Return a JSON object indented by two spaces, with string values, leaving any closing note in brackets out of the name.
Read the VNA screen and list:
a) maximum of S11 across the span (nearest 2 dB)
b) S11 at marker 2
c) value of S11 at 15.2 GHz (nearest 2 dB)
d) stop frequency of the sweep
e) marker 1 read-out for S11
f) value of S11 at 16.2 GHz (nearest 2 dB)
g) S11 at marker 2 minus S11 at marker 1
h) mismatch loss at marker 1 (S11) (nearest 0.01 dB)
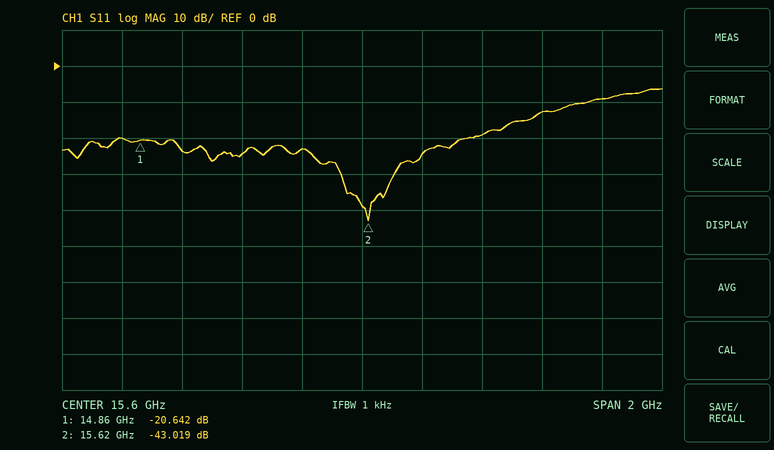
{
  "maximum of S11 across the span": "-6 dB",
  "S11 at marker 2": "-43.019 dB",
  "value of S11 at 15.2 GHz": "-24 dB",
  "stop frequency of the sweep": "16.6 GHz",
  "marker 1 read-out for S11": "-20.642 dB",
  "value of S11 at 16.2 GHz": "-12 dB",
  "S11 at marker 2 minus S11 at marker 1": "-22.377 dB",
  "mismatch loss at marker 1 (S11)": "0.04 dB"
}
